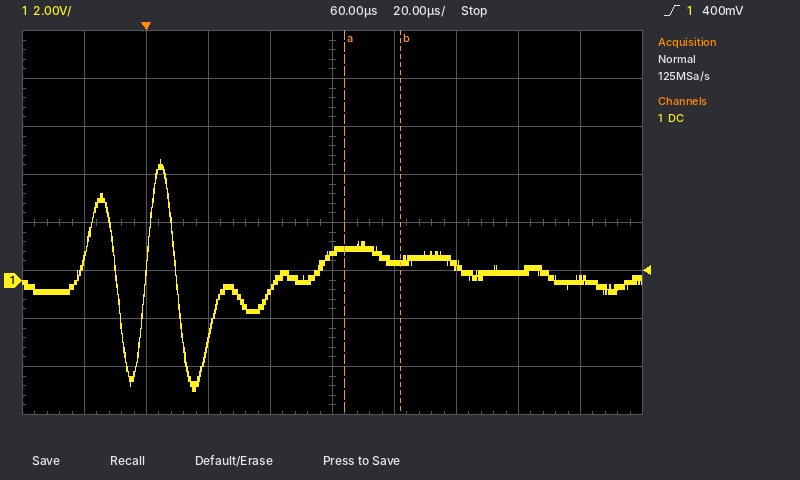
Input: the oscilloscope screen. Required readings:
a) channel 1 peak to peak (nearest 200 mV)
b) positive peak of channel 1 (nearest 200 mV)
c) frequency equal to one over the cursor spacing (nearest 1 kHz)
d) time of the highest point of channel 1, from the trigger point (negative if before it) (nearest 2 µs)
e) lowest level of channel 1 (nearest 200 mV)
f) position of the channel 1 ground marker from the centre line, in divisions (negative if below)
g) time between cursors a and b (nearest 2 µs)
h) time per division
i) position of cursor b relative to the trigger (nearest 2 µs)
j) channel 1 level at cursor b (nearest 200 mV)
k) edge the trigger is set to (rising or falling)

9.6 V
5.0 V
56 kHz
+4 µs
-4.6 V
-1.2 div
18 µs
20 µs
+82 µs
800 mV
rising
